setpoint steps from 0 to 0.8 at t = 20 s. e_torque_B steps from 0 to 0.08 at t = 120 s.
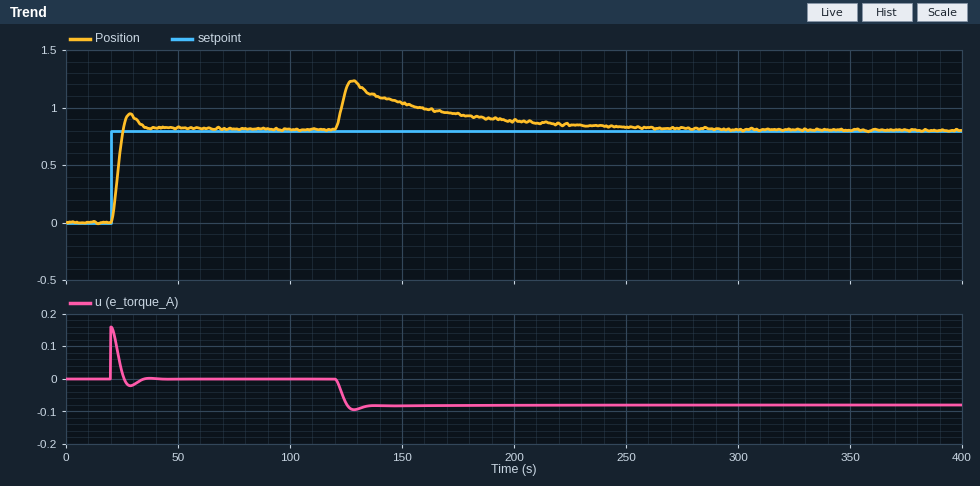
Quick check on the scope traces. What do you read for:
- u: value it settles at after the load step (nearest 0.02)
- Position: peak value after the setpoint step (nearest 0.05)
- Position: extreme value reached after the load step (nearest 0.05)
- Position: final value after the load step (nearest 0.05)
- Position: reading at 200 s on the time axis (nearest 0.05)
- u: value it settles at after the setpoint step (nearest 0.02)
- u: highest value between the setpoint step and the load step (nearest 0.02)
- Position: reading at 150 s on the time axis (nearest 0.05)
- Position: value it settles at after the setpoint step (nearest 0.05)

-0.08
0.95
1.25
0.80
0.90
0.00
0.16
1.05
0.80
